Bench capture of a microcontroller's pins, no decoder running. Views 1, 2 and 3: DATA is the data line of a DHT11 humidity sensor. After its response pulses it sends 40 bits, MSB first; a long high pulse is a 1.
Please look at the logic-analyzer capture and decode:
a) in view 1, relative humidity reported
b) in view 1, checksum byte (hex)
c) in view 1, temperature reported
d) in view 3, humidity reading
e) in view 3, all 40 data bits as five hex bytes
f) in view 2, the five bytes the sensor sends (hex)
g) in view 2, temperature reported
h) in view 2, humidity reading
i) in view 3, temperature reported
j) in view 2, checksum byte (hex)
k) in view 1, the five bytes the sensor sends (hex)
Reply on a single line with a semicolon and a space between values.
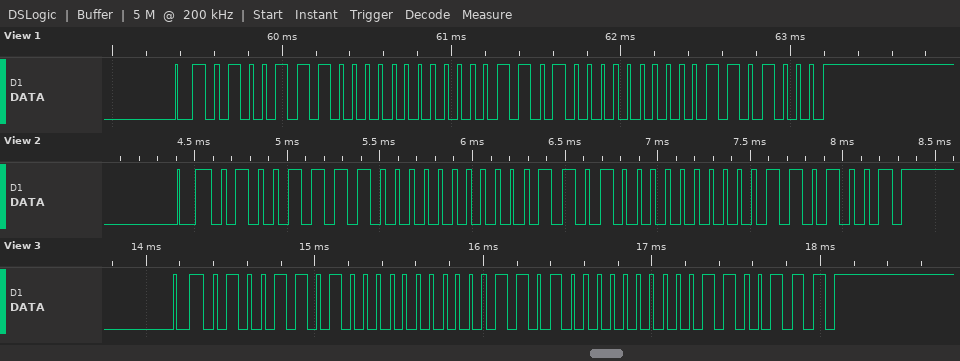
78 %; 0x68; 26.0 °C; 77 %; 4D 00 1A 00 67; 4F 00 1A 00 69; 26.0 °C; 79 %; 26.0 °C; 0x69; 4E 00 1A 00 68
